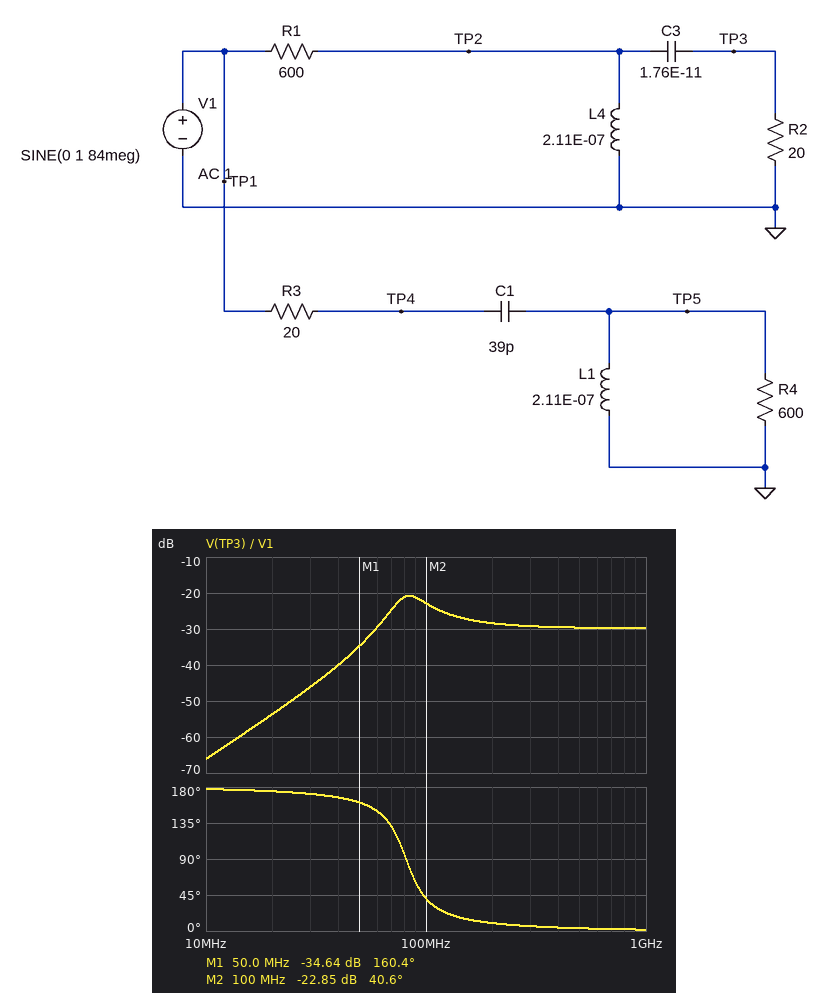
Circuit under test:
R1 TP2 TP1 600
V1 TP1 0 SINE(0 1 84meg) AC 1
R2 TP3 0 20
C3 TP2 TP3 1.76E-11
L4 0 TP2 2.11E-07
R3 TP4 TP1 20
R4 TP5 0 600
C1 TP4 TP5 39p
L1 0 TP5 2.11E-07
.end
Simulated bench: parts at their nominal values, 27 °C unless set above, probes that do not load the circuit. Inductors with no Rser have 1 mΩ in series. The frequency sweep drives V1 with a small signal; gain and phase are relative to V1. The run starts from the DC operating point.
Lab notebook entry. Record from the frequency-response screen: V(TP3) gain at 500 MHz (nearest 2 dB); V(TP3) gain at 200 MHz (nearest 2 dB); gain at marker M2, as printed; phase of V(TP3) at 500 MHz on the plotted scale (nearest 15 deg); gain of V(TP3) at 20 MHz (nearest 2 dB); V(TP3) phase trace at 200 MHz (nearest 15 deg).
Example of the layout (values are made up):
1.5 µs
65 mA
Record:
-30 dB
-28 dB
-22.85 dB
0 deg
-54 dB
15 deg
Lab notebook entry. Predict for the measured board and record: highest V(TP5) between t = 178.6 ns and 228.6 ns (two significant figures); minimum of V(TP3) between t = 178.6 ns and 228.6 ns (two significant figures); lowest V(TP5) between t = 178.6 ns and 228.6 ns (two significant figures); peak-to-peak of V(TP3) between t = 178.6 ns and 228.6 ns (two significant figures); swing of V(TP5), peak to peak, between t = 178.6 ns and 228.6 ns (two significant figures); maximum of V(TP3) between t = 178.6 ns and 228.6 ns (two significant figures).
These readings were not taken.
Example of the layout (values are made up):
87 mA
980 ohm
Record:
1.5 V
-91 mV
-1.5 V
180 mV
3.1 V
91 mV
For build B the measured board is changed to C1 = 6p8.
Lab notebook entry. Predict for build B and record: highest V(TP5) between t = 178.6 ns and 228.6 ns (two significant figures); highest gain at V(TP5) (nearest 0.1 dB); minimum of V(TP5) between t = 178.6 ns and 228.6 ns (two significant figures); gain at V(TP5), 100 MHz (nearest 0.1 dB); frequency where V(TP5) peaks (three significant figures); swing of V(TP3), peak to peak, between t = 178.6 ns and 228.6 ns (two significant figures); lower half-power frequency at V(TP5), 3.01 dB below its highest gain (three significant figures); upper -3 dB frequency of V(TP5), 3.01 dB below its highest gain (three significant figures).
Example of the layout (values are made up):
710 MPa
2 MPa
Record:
620 mV
7.8 dB
-620 mV
0.8 dB
136 MHz
180 mV
114 MHz
180 MHz
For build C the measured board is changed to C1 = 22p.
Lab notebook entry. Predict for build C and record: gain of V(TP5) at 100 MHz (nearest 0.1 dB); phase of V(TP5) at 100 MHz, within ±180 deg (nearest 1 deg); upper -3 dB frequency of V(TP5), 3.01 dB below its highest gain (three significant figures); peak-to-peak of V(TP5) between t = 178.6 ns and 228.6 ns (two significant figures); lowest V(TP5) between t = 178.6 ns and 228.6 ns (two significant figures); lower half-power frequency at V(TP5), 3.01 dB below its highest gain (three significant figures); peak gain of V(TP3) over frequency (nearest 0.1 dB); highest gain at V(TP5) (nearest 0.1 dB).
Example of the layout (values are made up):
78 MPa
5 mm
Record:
5.1 dB
29 deg
95.5 MHz
4.8 V
-2.4 V
64.0 MHz
-20.8 dB
8.7 dB
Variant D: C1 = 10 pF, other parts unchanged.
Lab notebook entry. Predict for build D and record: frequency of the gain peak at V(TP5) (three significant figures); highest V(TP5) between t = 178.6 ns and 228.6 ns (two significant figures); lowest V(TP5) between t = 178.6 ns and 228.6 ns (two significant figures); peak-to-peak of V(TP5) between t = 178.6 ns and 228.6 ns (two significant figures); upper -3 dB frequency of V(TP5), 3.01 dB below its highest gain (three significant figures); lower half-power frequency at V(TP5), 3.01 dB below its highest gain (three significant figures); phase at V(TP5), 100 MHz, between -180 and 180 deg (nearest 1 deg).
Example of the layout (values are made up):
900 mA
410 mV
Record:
112 MHz
1.2 V
-1.2 V
2.4 V
144 MHz
94.6 MHz
112 deg
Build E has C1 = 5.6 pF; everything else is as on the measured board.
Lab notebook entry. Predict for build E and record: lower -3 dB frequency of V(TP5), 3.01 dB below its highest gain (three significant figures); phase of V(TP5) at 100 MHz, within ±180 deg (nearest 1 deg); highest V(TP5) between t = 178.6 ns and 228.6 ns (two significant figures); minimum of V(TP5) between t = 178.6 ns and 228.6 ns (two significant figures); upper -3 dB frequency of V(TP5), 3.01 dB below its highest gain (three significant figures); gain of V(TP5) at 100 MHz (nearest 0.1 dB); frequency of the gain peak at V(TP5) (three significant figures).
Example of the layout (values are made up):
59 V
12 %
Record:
125 MHz
151 deg
470 mV
-470 mV
203 MHz
-2.1 dB
151 MHz
